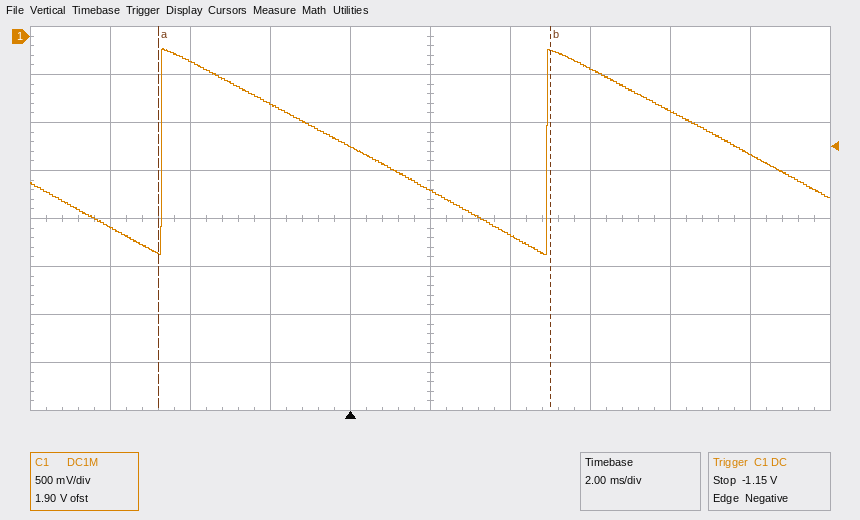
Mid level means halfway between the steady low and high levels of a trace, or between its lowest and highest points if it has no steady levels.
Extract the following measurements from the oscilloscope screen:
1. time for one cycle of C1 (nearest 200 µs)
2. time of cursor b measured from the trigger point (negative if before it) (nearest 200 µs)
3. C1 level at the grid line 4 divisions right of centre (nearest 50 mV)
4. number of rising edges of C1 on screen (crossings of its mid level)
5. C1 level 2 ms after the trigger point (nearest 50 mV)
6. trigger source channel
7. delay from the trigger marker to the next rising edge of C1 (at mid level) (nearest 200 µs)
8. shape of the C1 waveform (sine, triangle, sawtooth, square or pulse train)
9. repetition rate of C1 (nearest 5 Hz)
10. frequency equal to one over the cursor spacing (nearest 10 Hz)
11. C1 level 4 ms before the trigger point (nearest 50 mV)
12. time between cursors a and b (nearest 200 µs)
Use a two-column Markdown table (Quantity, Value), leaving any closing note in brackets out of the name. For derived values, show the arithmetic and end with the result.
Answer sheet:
| Quantity | Value |
|---|---|
| time for one cycle of C1 | 9.6 ms |
| time of cursor b measured from the trigger point (negative if before it) | +5.0 ms |
| C1 level at the grid line 4 divisions right of centre | -1.25 V |
| number of rising edges of C1 on screen | 2 |
| C1 level 2 ms after the trigger point | -1.60 V |
| trigger source channel | C1 |
| delay from the trigger marker to the next rising edge of C1 (at mid level) | 5.0 ms |
| shape of the C1 waveform | sawtooth |
| repetition rate of C1 | 1 / 9.6 ms ≈ 104 Hz, so 105 Hz to the nearest 5 Hz |
| frequency equal to one over the cursor spacing | 1 / 9.8 ms ≈ 100 Hz |
| C1 level 4 ms before the trigger point | -250 mV |
| time between cursors a and b | 9.8 ms |
